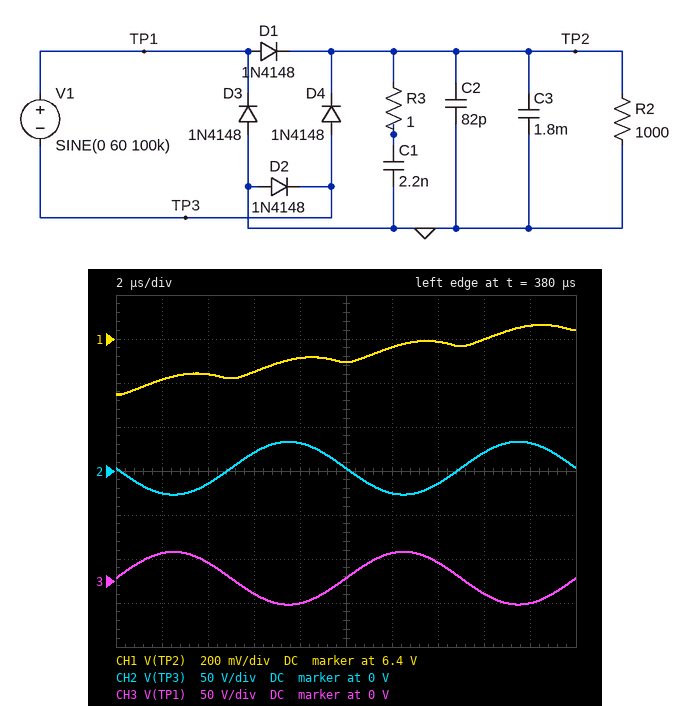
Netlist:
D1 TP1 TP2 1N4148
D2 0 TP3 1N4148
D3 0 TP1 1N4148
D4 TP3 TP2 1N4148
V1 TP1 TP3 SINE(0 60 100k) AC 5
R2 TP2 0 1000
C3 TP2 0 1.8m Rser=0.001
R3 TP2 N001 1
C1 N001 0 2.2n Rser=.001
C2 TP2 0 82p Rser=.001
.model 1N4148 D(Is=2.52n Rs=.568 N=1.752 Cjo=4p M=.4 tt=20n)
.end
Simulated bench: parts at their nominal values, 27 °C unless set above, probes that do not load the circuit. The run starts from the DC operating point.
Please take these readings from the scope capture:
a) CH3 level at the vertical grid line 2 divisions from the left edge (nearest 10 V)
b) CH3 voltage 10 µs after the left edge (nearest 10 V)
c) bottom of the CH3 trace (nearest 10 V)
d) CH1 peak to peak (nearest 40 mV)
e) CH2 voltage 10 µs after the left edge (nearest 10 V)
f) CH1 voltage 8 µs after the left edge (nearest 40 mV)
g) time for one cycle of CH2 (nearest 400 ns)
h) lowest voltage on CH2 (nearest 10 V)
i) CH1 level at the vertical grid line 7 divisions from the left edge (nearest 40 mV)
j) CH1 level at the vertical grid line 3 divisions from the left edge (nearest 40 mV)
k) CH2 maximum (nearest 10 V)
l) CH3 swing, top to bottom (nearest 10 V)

20 V
0 V
-30 V
320 mV
0 V
6.32 V
10.0 µs
-30 V
6.40 V
6.24 V
30 V
60 V
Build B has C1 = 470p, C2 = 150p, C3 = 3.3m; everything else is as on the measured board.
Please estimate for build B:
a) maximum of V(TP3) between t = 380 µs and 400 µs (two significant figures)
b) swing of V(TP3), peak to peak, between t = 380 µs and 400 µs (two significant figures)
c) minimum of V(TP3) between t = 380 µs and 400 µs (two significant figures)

32 V
60 V
-28 V
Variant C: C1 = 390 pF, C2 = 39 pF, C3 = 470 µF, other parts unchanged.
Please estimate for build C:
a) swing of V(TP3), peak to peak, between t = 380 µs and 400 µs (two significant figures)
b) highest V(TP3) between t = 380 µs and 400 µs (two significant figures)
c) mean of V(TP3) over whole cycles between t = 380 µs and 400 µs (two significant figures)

60 V
40 V
9.7 V
